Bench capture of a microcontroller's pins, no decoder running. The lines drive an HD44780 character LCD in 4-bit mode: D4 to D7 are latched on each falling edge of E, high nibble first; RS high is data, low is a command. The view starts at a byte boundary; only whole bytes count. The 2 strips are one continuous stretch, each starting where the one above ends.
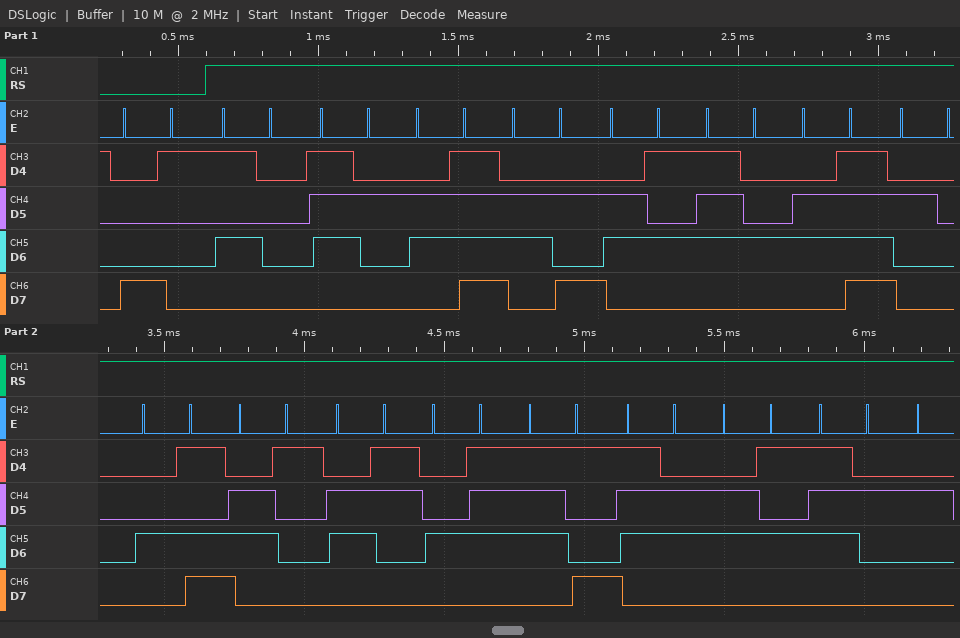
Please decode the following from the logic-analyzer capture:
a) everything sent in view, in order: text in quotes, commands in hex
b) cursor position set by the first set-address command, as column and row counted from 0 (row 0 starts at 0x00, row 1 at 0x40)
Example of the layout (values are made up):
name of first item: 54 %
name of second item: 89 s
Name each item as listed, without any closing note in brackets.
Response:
everything sent in view, in order: text in quotes, commands in hex: 0x81 "Projeto MacGyver"
cursor position set by the first set-address command, as column and row counted from 0: column 1, row 0
